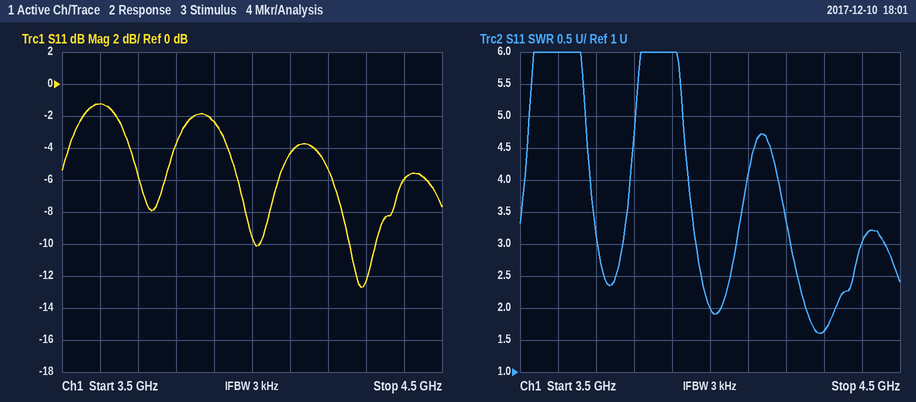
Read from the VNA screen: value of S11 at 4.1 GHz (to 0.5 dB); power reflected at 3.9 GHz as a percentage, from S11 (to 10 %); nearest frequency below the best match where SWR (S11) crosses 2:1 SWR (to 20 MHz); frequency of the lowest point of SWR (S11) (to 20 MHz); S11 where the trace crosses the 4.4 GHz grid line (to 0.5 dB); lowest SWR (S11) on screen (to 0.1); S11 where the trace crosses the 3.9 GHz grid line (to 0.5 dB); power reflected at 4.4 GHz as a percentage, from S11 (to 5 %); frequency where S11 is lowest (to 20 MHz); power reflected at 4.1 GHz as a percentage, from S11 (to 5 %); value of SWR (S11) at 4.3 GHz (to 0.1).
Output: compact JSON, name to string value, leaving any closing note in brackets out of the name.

{"value of S11 at 4.1 GHz": "-4.5 dB", "power reflected at 3.9 GHz as a percentage, from S11": "60 %", "nearest frequency below the best match where SWR (S11) crosses 2:1 SWR": "4.26 GHz", "frequency of the lowest point of SWR (S11)": "4.28 GHz", "S11 where the trace crosses the 4.4 GHz grid line": "-6.0 dB", "lowest SWR (S11) on screen": "1.6", "S11 where the trace crosses the 3.9 GHz grid line": "-2.5 dB", "power reflected at 4.4 GHz as a percentage, from S11": "25 %", "frequency where S11 is lowest": "4.28 GHz", "power reflected at 4.1 GHz as a percentage, from S11": "35 %", "value of SWR (S11) at 4.3 GHz": "1.6"}
